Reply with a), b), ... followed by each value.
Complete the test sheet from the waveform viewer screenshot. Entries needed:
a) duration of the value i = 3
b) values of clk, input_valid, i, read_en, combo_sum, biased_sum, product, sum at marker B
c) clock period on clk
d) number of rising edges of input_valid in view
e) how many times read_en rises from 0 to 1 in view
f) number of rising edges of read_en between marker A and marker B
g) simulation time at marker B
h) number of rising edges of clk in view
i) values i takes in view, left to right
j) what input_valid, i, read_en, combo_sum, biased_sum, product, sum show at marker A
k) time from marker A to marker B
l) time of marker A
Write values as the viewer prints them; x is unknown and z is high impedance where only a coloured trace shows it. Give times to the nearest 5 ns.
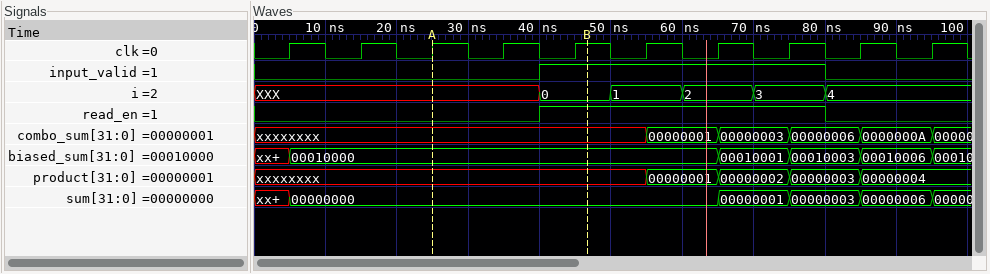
a) 10 ns
b) clk=1, input_valid=1, i=0, read_en=1, combo_sum=xxxxxxxx, biased_sum=00010000, product=xxxxxxxx, sum=00000000
c) 10 ns
d) 1
e) 1
f) 1
g) 45 ns
h) 10
i) XXX, 0, 1, 2, 3, 4
j) input_valid=0, i=XXX, read_en=0, combo_sum=xxxxxxxx, biased_sum=00010000, product=xxxxxxxx, sum=00000000
k) 20 ns
l) 25 ns
